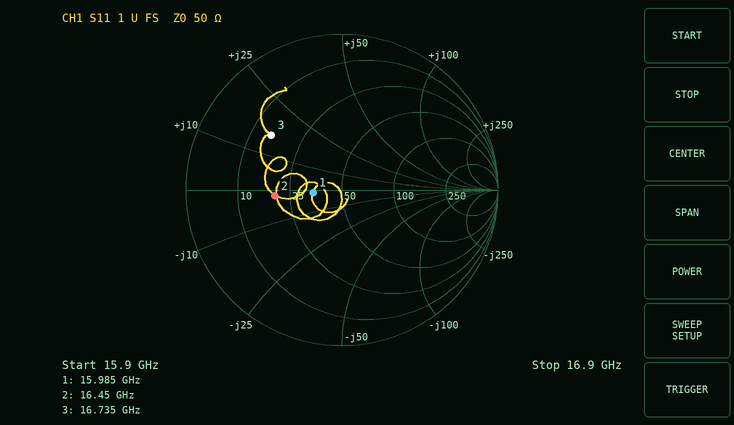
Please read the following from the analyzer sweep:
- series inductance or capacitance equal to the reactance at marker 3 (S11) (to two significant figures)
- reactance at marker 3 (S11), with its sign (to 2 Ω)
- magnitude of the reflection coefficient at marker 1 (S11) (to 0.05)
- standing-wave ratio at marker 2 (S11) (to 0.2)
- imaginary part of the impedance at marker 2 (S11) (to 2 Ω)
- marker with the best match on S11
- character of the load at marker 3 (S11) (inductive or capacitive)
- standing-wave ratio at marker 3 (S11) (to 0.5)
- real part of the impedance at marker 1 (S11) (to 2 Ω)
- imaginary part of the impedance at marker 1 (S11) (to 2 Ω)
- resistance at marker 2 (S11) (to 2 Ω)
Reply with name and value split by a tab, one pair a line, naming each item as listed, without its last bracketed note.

series inductance or capacitance equal to the reactance at marker 3 (S11)	150 pH
reactance at marker 3 (S11), with its sign	+16 Ω
magnitude of the reflection coefficient at marker 1 (S11)	0.20
standing-wave ratio at marker 2 (S11)	2.6
imaginary part of the impedance at marker 2 (S11)	-2 Ω
marker with the best match on S11	marker 1
character of the load at marker 3 (S11)	inductive
standing-wave ratio at marker 3 (S11)	3.5
real part of the impedance at marker 1 (S11)	34 Ω
imaginary part of the impedance at marker 1 (S11)	-2 Ω
resistance at marker 2 (S11)	20 Ω
